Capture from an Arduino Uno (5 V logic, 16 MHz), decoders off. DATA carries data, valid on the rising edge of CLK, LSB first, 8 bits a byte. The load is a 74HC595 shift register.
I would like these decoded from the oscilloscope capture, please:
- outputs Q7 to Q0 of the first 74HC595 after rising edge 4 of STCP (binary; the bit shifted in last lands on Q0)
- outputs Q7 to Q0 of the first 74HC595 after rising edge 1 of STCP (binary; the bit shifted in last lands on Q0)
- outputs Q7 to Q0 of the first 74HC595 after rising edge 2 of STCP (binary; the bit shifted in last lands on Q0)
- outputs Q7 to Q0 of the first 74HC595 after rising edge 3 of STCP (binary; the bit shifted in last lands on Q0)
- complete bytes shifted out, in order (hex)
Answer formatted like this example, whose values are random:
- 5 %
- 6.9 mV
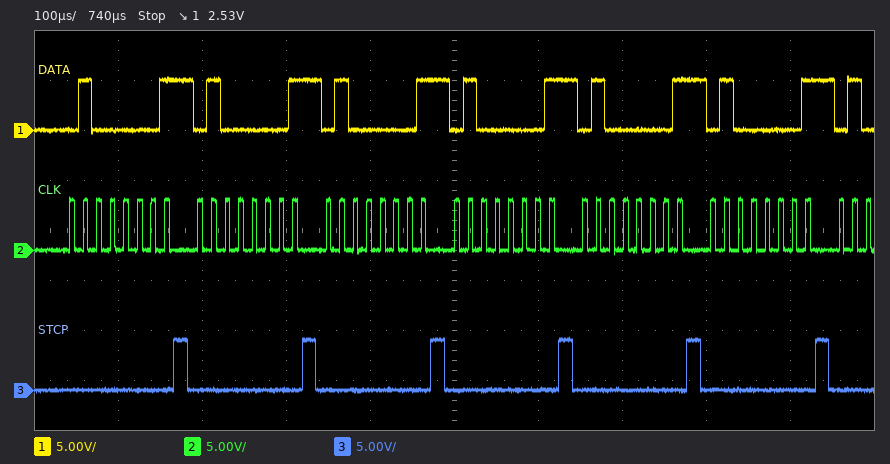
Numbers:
- 01000001
- 01000001
- 01000001
- 01000001
- 82 82 82 82 82 82
